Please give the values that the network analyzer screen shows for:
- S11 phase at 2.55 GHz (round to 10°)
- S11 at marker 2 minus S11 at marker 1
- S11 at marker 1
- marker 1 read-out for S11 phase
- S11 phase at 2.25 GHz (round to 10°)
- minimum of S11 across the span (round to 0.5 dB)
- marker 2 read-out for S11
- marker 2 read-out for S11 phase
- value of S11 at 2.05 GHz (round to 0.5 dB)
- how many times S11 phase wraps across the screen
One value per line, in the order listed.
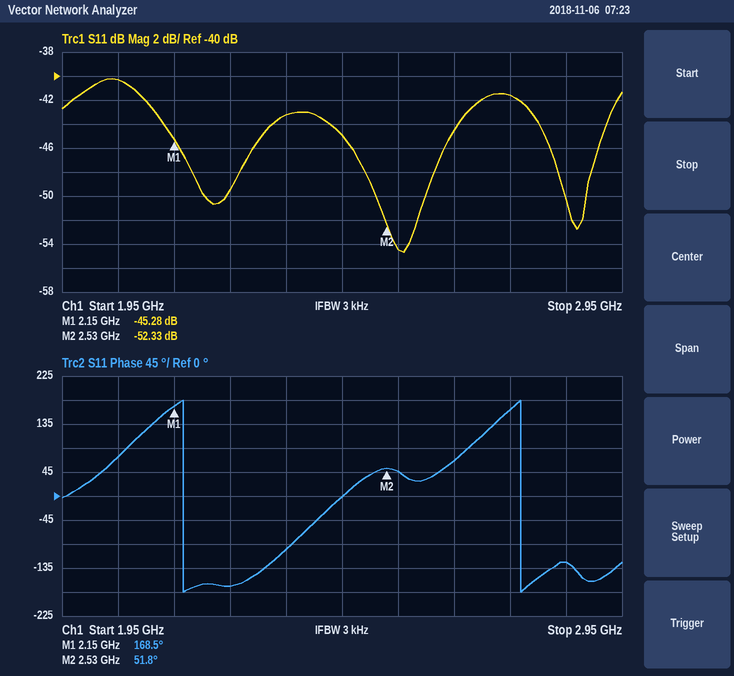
50°
-7.05 dB
-45.28 dB
168.5°
-170°
-54.5 dB
-52.33 dB
51.8°
-40.5 dB
2
